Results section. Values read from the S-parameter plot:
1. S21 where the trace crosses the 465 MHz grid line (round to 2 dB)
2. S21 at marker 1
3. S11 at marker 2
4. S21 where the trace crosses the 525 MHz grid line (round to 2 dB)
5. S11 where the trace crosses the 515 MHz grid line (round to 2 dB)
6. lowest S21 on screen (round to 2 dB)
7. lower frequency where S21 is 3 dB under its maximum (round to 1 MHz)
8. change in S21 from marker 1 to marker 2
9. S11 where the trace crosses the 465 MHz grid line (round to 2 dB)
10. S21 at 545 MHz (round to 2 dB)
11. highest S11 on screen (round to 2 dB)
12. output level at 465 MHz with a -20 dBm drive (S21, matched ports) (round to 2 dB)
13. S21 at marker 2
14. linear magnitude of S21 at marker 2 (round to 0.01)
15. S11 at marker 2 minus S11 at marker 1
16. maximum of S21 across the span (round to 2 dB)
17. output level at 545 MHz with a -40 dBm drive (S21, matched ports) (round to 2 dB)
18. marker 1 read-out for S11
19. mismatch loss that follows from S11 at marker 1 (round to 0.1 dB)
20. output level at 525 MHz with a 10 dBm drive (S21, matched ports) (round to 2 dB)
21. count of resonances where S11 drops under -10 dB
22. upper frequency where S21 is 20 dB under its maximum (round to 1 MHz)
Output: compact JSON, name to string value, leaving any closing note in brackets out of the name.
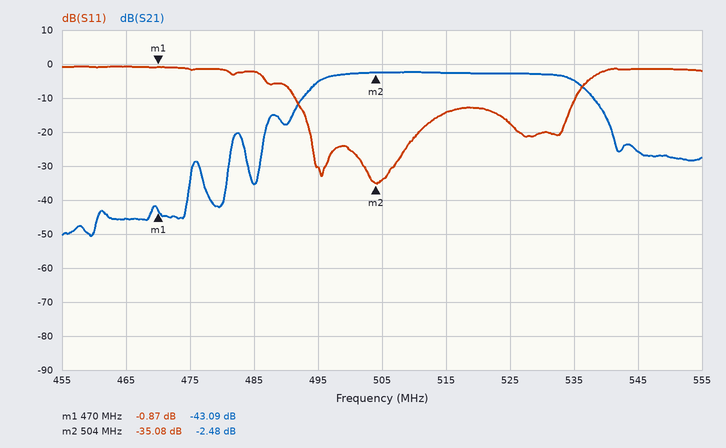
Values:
{"S21 where the trace crosses the 465 MHz grid line": "-46 dB", "S21 at marker 1": "-43.09 dB", "S11 at marker 2": "-35.08 dB", "S21 where the trace crosses the 525 MHz grid line": "-2 dB", "S11 where the trace crosses the 515 MHz grid line": "-14 dB", "lowest S21 on screen": "-50 dB", "lower frequency where S21 is 3 dB under its maximum": "495 MHz", "change in S21 from marker 1 to marker 2": "40.61 dB", "S11 where the trace crosses the 465 MHz grid line": "0 dB", "S21 at 545 MHz": "-26 dB", "highest S11 on screen": "0 dB", "output level at 465 MHz with a -20 dBm drive (S21, matched ports)": "-66 dBm", "S21 at marker 2": "-2.48 dB", "linear magnitude of S21 at marker 2": "0.75", "S11 at marker 2 minus S11 at marker 1": "-34.21 dB", "maximum of S21 across the span": "-2 dB", "output level at 545 MHz with a -40 dBm drive (S21, matched ports)": "-66 dBm", "marker 1 read-out for S11": "-0.87 dB", "mismatch loss that follows from S11 at marker 1": "7.4 dB", "output level at 525 MHz with a 10 dBm drive (S21, matched ports)": "8 dBm", "count of resonances where S11 drops under -10 dB": "3", "upper frequency where S21 is 20 dB under its maximum": "541 MHz"}
